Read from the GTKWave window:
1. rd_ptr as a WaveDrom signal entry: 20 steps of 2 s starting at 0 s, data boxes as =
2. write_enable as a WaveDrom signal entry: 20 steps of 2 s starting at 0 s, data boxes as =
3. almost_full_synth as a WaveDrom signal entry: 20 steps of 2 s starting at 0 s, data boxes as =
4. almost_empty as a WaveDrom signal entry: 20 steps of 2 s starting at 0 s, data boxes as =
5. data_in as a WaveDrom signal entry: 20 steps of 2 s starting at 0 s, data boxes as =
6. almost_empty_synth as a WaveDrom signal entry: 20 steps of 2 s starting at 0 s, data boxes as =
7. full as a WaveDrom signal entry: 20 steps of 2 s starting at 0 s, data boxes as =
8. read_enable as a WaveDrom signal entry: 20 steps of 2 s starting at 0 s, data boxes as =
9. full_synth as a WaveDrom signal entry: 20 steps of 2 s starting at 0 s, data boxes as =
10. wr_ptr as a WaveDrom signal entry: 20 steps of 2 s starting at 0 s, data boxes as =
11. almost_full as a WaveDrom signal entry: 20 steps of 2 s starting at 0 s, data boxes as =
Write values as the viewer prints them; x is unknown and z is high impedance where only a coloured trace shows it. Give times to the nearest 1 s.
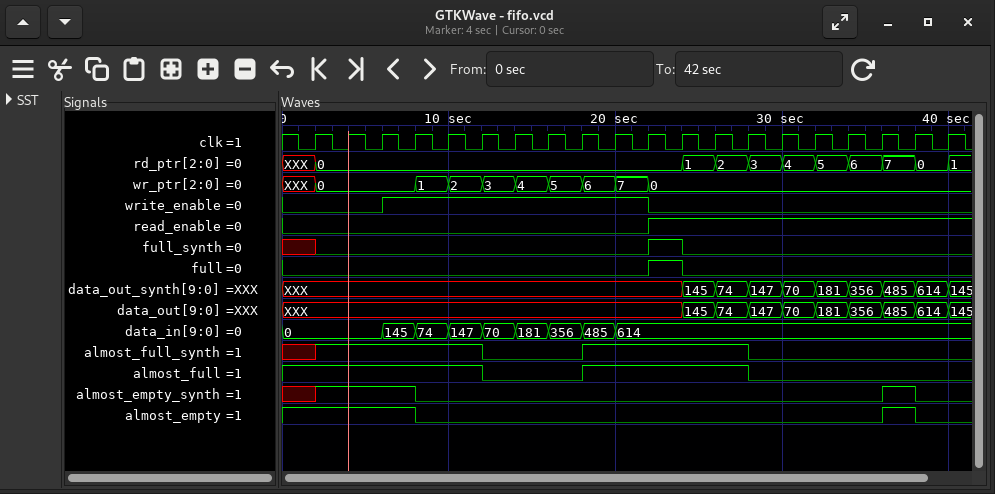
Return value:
{name: 'rd_ptr', wave: 'x=..........========', data: '0 1 2 3 4 5 6 7 0'}
{name: 'write_enable', wave: '0..1.......0........'}
{name: 'almost_full_synth', wave: 'x1....0..1....0.....'}
{name: 'almost_empty', wave: '1...0.............10'}
{name: 'data_in', wave: '=..========.........', data: '0 145 74 147 70 181 356 485 614'}
{name: 'almost_empty_synth', wave: 'x1..0.............10'}
{name: 'full', wave: '0..........10.......'}
{name: 'read_enable', wave: '0..........1........'}
{name: 'full_synth', wave: 'x0.........10.......'}
{name: 'wr_ptr', wave: 'x=..========........', data: '0 1 2 3 4 5 6 7 0'}
{name: 'almost_full', wave: '1.....0..1....0.....'}
